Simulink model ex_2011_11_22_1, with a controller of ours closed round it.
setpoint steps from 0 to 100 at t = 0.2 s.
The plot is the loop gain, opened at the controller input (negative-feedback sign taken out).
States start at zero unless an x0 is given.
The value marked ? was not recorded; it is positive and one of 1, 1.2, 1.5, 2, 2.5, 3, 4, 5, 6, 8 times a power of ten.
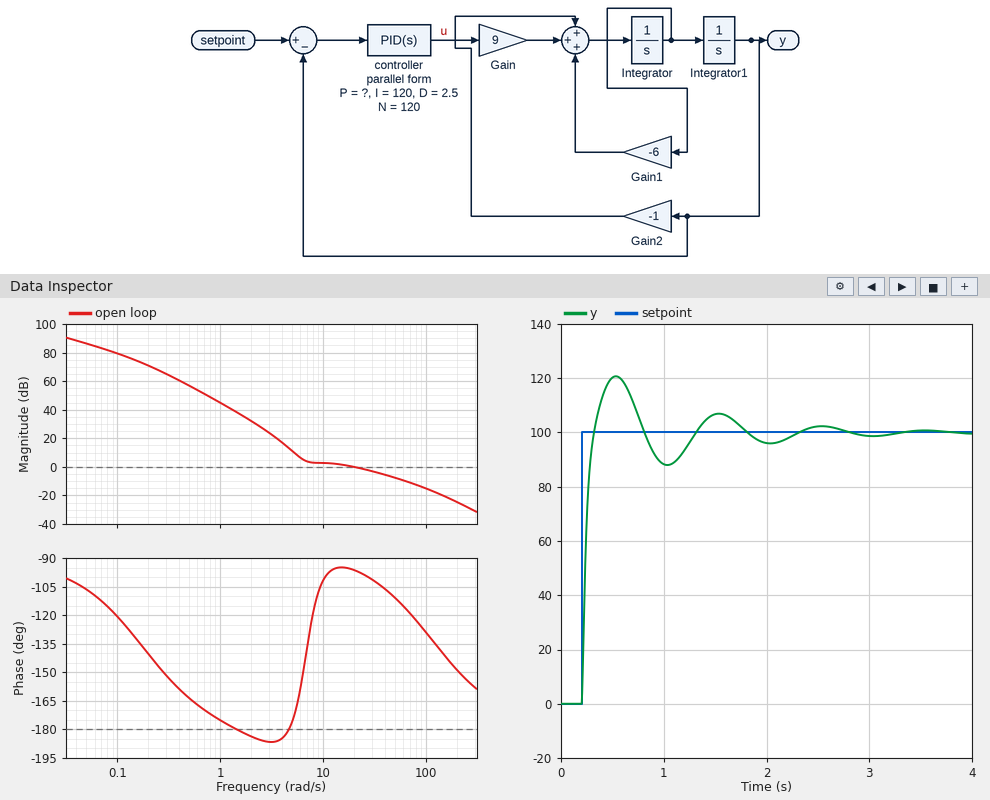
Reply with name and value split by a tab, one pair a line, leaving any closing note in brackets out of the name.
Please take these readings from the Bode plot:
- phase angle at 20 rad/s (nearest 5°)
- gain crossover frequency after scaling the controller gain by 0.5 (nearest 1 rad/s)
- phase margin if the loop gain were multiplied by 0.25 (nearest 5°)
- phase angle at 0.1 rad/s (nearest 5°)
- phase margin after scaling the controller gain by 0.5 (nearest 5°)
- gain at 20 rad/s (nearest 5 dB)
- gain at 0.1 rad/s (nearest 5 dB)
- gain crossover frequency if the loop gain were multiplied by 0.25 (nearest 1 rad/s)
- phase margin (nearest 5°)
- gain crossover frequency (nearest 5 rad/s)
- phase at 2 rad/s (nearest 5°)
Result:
phase angle at 20 rad/s	-95°
gain crossover frequency after scaling the controller gain by 0.5	6 rad/s
phase margin if the loop gain were multiplied by 0.25	0°
phase angle at 0.1 rad/s	-120°
phase margin after scaling the controller gain by 0.5	25°
gain at 20 rad/s	0 dB
gain at 0.1 rad/s	80 dB
gain crossover frequency if the loop gain were multiplied by 0.25	5 rad/s
phase margin	85°
gain crossover frequency	20 rad/s
phase at 2 rad/s	-185°
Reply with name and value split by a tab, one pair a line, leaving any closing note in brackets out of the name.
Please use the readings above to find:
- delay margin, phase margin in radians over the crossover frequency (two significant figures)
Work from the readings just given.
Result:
delay margin, phase margin in radians over the crossover frequency	0.074 s
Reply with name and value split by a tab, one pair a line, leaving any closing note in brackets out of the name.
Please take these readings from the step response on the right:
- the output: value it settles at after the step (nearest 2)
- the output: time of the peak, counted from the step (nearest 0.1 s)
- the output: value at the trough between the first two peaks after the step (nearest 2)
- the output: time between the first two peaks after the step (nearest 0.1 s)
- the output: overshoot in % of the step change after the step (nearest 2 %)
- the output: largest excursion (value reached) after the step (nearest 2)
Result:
the output: value it settles at after the step	100
the output: time of the peak, counted from the step	0.3 s
the output: value at the trough between the first two peaks after the step	88
the output: time between the first two peaks after the step	1.0 s
the output: overshoot in % of the step change after the step	20 %
the output: largest excursion (value reached) after the step	120
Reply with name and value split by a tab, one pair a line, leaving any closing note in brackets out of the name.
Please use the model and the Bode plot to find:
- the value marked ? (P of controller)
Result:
the value marked ?	10
